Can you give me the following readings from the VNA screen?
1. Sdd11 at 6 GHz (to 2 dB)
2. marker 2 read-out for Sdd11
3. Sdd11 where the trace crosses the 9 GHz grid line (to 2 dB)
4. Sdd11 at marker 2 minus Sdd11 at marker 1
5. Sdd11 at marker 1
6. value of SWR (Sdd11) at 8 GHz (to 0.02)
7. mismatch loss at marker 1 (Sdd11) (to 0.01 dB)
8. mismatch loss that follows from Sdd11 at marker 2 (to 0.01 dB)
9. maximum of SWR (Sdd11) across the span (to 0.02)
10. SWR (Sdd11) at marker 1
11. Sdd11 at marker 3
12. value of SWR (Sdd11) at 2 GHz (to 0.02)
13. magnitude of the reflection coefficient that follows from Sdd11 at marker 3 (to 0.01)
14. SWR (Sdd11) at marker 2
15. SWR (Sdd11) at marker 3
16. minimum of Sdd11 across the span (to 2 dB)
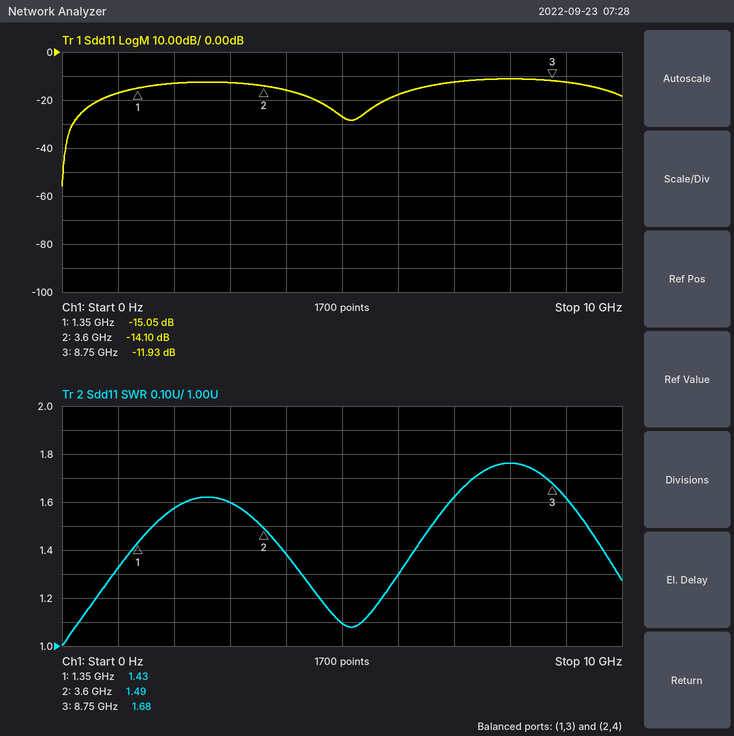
-18 dB
-14.10 dB
-12 dB
0.95 dB
-15.05 dB
1.76
0.14 dB
0.17 dB
1.76
1.43
-11.93 dB
1.58
0.25
1.49
1.68
-56 dB
